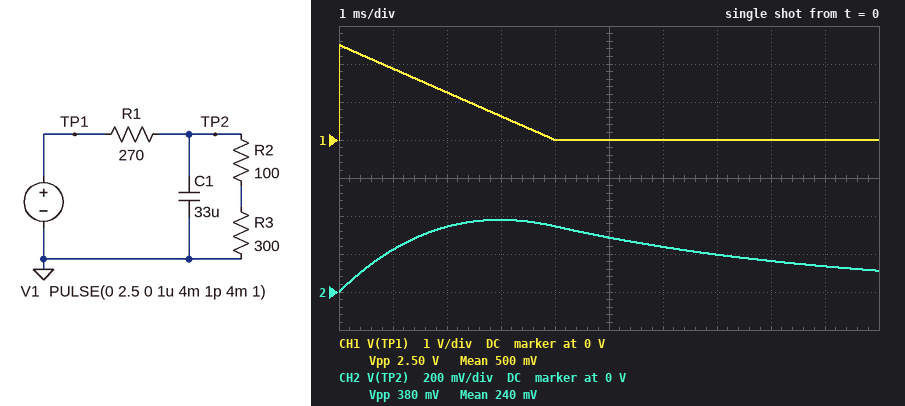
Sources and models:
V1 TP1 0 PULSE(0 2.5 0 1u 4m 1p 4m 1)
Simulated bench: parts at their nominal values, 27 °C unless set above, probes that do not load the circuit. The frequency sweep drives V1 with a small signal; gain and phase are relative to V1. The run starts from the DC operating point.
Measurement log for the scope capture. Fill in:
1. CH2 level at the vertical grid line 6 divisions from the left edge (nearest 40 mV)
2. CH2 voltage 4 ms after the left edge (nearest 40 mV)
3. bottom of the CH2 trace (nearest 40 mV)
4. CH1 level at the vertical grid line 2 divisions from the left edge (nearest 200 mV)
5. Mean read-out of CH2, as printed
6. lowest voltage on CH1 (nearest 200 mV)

240 mV
360 mV
0 V
1.2 V
240 mV
0 V
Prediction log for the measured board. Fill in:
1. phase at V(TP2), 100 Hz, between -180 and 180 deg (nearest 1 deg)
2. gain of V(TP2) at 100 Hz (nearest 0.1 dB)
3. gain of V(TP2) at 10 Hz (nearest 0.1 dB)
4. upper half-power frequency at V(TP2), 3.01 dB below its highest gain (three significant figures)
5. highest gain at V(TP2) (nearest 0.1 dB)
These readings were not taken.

-73 deg
-15.3 dB
-4.9 dB
29.9 Hz
-4.5 dB
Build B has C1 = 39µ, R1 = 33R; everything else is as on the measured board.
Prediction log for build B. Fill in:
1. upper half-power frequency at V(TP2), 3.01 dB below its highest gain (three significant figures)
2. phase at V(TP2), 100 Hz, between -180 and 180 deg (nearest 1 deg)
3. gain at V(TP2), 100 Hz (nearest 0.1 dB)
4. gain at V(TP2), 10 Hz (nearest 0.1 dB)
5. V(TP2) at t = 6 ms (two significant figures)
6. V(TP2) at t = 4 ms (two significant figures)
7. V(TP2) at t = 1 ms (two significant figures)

134 Hz
-37 deg
-2.6 dB
-0.7 dB
110 mV
580 mV
1.1 V
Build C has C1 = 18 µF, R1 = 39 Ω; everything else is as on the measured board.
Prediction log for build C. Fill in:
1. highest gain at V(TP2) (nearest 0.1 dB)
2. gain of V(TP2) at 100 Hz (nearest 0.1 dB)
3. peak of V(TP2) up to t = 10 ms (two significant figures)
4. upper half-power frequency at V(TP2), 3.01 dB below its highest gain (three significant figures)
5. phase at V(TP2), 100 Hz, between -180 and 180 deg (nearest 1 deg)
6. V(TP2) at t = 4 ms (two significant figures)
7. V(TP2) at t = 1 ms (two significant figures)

-0.8 dB
-1.5 dB
1.6 V
249 Hz
-22 deg
360 mV
1.5 V
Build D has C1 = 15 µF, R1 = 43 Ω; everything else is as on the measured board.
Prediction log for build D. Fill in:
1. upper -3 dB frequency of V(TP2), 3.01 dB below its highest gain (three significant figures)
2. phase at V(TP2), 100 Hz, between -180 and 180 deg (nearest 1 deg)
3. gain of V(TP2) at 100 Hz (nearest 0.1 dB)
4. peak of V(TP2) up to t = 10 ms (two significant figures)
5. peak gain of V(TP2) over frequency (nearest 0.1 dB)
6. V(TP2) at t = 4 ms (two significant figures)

273 Hz
-20 deg
-1.4 dB
1.6 V
-0.9 dB
330 mV
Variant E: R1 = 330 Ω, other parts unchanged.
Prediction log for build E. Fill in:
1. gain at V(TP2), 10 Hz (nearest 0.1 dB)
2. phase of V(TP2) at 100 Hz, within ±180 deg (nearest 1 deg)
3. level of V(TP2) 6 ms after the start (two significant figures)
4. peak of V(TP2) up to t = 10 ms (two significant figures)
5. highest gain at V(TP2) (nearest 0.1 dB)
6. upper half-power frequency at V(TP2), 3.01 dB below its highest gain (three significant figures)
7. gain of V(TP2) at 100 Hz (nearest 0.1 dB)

-5.8 dB
-75 deg
210 mV
320 mV
-5.2 dB
26.7 Hz
-17.0 dB
